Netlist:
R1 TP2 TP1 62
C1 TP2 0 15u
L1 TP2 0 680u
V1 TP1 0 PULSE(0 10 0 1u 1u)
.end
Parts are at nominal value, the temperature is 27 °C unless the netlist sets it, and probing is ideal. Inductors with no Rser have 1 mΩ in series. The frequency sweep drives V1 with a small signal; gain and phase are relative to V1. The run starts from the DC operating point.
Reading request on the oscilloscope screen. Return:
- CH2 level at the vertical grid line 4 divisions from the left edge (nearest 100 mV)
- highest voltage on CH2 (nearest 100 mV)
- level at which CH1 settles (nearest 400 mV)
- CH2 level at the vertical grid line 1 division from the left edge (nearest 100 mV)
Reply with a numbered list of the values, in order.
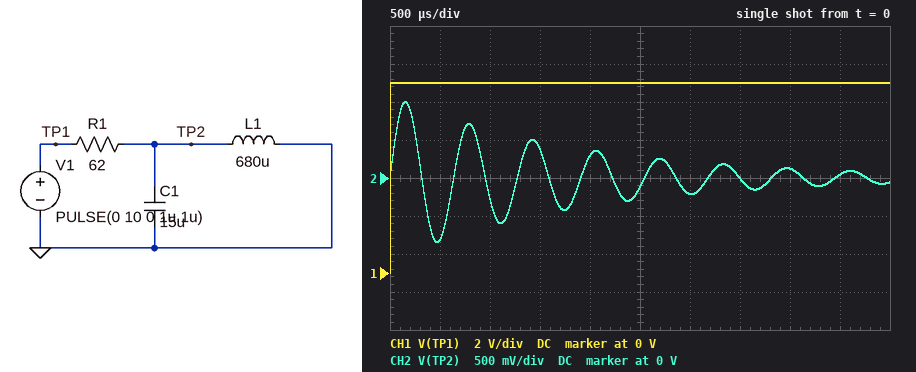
1. 300 mV
2. 1.0 V
3. 10.0 V
4. -800 mV
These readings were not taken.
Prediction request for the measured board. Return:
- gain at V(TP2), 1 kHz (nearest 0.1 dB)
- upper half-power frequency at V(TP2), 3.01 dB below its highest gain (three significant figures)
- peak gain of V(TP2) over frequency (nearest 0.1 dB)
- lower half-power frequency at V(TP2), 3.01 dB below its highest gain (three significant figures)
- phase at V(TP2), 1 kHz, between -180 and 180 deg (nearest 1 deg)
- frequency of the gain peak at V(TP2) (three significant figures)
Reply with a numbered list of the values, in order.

1. -18.8 dB
2. 1.66 kHz
3. 0 dB
4. 1.49 kHz
5. 83 deg
6. 1.58 kHz
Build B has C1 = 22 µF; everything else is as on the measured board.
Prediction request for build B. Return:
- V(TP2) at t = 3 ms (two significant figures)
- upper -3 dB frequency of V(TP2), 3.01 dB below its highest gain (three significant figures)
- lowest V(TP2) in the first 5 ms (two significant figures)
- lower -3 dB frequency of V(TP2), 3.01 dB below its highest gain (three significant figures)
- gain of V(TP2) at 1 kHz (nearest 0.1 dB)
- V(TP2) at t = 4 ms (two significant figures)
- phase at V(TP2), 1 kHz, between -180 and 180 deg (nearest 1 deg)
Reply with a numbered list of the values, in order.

1. -180 mV
2. 1.36 kHz
3. -730 mV
4. 1.24 kHz
5. -15.6 dB
6. 200 mV
7. 80 deg
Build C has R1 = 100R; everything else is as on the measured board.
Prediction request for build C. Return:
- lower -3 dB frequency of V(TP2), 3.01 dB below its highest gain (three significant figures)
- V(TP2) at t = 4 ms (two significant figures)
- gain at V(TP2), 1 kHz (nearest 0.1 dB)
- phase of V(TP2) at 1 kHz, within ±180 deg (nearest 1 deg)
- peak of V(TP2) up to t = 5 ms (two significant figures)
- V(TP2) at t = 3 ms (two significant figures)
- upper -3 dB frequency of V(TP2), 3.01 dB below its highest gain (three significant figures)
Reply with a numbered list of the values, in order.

1. 1.52 kHz
2. 170 mV
3. -22.9 dB
4. 86 deg
5. 640 mV
6. -240 mV
7. 1.63 kHz
